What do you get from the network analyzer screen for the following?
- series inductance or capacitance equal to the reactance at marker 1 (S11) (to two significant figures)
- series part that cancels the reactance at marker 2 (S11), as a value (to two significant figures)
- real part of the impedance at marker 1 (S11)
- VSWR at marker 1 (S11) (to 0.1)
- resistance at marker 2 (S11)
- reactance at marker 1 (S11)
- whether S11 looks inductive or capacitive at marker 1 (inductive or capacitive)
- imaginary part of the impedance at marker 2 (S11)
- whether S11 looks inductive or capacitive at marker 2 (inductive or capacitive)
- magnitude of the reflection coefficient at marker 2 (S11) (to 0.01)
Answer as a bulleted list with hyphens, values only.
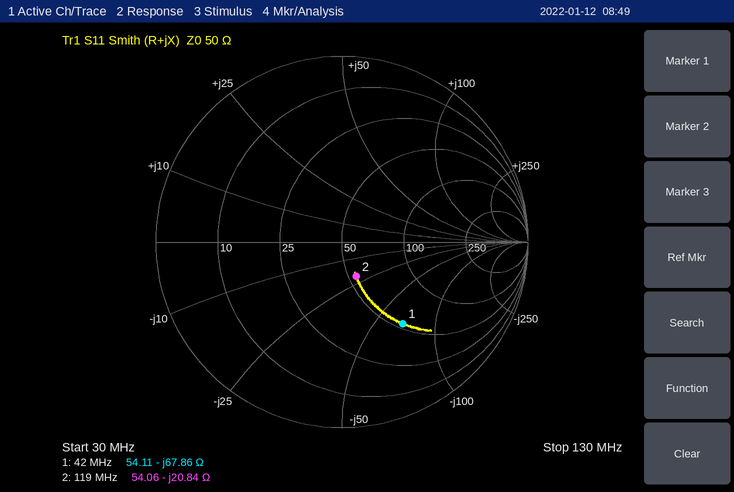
- 56 pF
- 28 nH
- 54.11 Ω
- 3.4
- 54.06 Ω
- -67.86 Ω
- capacitive
- -20.84 Ω
- capacitive
- 0.20
